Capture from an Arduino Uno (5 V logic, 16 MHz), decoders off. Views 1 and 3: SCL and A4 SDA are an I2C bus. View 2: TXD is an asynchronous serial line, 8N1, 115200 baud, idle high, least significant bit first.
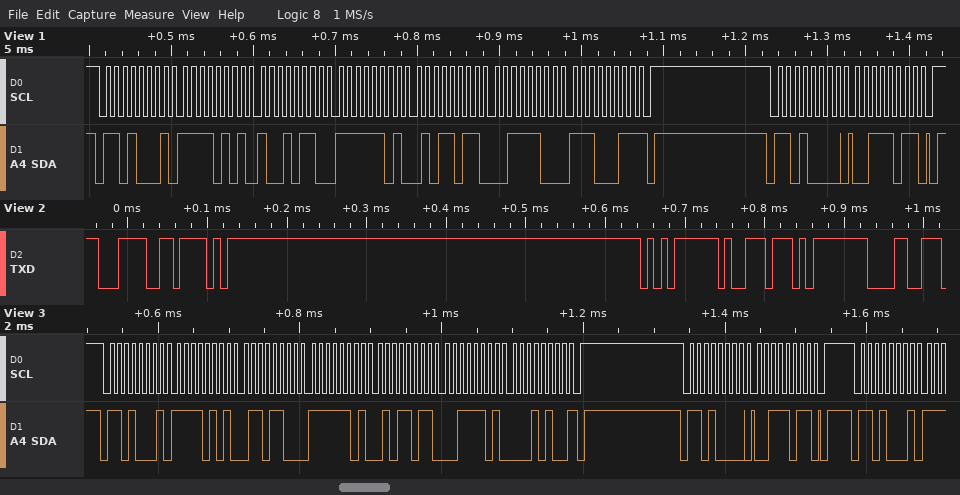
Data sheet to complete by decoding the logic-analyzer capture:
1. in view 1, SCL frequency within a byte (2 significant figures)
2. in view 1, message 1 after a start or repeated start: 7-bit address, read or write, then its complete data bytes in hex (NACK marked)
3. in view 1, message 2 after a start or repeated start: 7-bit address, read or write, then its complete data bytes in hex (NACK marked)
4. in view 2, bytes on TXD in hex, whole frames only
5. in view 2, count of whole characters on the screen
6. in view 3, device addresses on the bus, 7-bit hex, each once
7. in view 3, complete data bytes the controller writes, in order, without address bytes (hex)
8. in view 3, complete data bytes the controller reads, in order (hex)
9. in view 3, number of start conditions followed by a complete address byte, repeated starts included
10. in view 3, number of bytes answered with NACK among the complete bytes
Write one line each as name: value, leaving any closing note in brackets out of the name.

in view 1, SCL frequency within a byte: 100 kHz
in view 1, message 1 after a start or repeated start: 7-bit address, read or write, then its complete data bytes in hex: 0x68 read: F5 96 FD 5B 3C E3 NACK
in view 1, message 2 after a start or repeated start: 7-bit address, read or write, then its complete data bytes in hex: 0x68 write: 3B
in view 2, bytes on TXD in hex, whole frames only: 3C AF F5 B9 FD 98
in view 2, count of whole characters on the screen: 6
in view 3, device addresses on the bus, 7-bit hex, each once: 0x68
in view 3, complete data bytes the controller writes, in order, without address bytes: 3B
in view 3, complete data bytes the controller reads, in order: F5 6C FD 5B 3D 14
in view 3, number of start conditions followed by a complete address byte, repeated starts included: 3
in view 3, number of bytes answered with NACK among the complete bytes: 1
